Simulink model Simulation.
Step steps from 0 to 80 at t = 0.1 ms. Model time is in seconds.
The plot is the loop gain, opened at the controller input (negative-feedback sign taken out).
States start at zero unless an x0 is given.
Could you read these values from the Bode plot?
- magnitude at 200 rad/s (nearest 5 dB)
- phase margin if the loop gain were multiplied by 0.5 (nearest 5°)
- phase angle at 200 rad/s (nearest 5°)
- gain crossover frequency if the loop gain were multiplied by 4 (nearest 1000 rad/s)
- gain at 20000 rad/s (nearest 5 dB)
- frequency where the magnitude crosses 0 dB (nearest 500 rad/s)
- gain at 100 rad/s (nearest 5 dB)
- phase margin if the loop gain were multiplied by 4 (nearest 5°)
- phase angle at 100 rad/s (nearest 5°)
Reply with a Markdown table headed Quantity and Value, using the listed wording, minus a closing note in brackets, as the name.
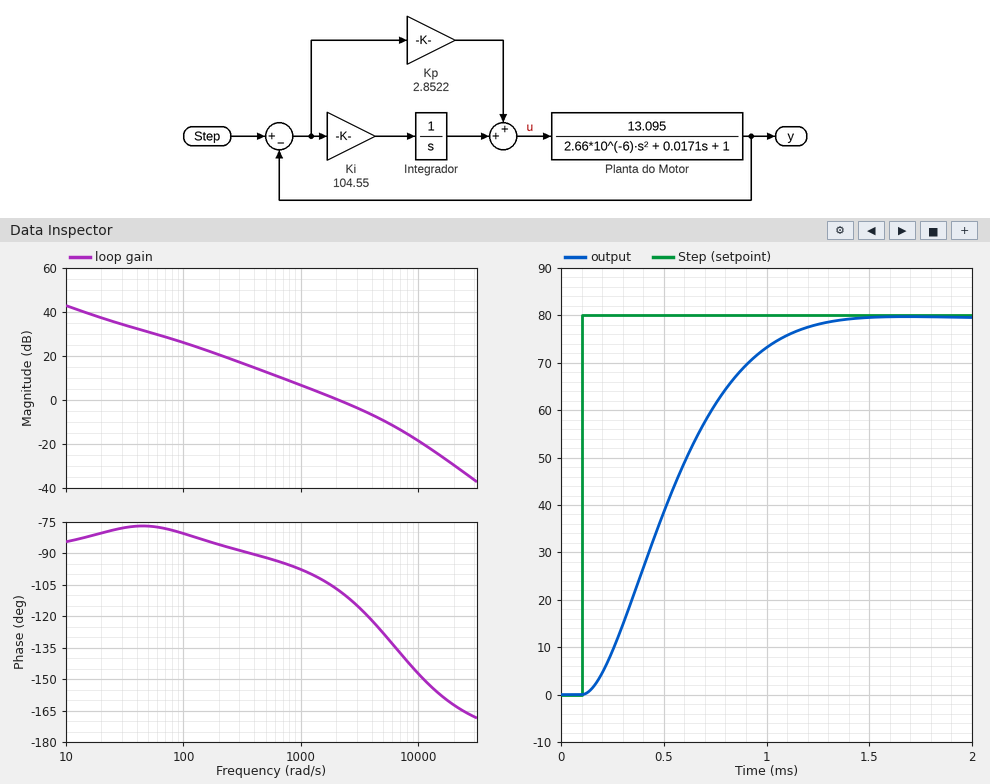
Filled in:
| Quantity | Value |
|---|---|
| magnitude at 200 rad/s | 20 dB |
| phase margin if the loop gain were multiplied by 0.5 | 80° |
| phase angle at 200 rad/s | -85° |
| gain crossover frequency if the loop gain were multiplied by 4 | 6000 rad/s |
| gain at 20000 rad/s | -30 dB |
| frequency where the magnitude crosses 0 dB | 2000 rad/s |
| gain at 100 rad/s | 25 dB |
| phase margin if the loop gain were multiplied by 4 | 45° |
| phase angle at 100 rad/s | -80° |
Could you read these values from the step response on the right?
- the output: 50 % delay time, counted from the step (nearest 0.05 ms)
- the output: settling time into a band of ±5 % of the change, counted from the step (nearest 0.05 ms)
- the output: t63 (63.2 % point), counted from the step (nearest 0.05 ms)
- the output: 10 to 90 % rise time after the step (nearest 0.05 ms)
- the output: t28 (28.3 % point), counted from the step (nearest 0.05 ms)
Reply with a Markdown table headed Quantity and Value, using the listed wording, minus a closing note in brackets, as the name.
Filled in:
| Quantity | Value |
|---|---|
| the output: 50 % delay time, counted from the step | 0.40 ms |
| the output: settling time into a band of ±5 % of the change, counted from the step | 1.00 ms |
| the output: t63 (63.2 % point), counted from the step | 0.50 ms |
| the output: 10 to 90 % rise time after the step | 0.70 ms |
| the output: t28 (28.3 % point), counted from the step | 0.25 ms |
